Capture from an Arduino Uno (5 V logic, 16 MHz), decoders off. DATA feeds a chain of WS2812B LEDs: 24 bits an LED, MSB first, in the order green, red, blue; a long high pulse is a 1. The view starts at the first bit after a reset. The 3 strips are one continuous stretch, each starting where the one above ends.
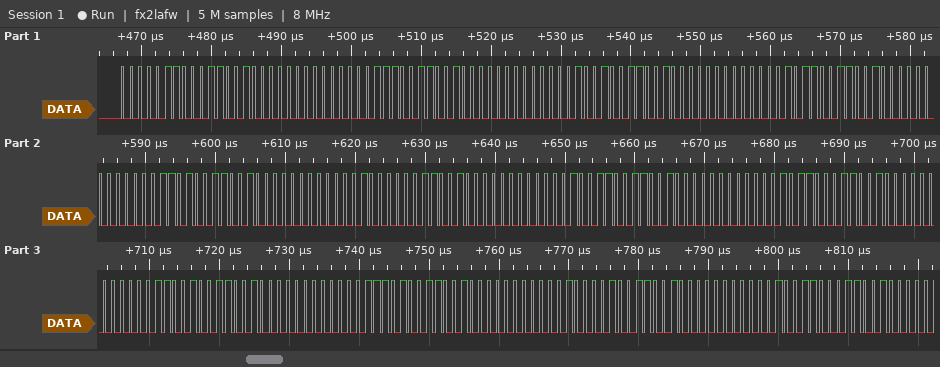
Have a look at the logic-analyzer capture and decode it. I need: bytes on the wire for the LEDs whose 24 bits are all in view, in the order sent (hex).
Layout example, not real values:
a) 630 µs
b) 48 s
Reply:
a) 06 32 00 07 32 00 09 32 00 0B 32 00 0D 32 00 10 32 00 13 32 00 16 32 00 19 32 00 1D 32 00 21 32 00
